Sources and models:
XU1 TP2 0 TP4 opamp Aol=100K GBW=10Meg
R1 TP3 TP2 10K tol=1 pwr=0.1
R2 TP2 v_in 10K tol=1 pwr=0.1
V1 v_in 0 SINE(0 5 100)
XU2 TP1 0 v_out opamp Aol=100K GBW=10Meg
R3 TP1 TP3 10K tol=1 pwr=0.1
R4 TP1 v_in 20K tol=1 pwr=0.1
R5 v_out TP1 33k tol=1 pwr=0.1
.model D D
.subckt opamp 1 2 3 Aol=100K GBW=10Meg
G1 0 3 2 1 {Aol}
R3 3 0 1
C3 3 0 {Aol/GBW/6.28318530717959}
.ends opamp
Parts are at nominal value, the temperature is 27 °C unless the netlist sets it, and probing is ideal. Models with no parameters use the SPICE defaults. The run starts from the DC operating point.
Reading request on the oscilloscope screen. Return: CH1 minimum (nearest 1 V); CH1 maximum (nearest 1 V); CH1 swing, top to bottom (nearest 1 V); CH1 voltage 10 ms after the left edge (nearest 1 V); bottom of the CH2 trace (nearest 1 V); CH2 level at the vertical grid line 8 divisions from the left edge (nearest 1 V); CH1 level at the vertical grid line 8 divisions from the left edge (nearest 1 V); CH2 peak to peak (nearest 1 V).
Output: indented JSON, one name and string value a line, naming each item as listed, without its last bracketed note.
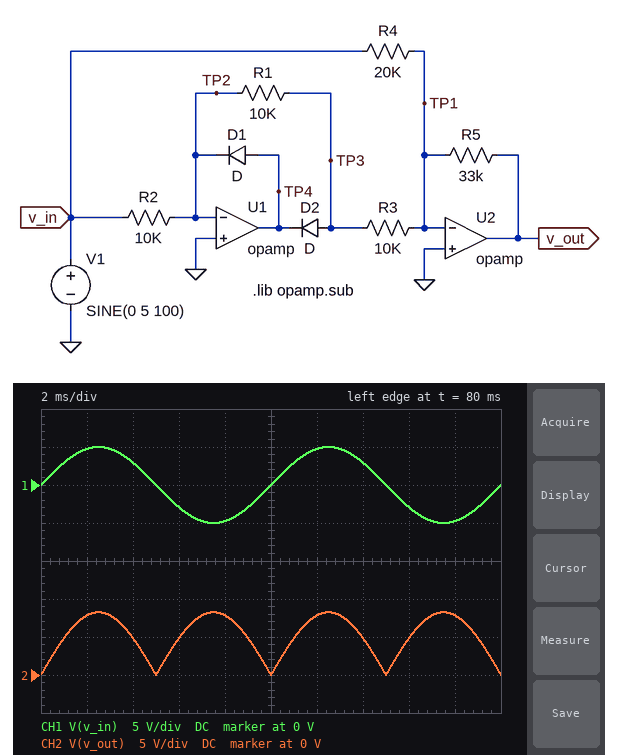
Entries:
{
  "CH1 minimum": "-5 V",
  "CH1 maximum": "5 V",
  "CH1 swing, top to bottom": "10 V",
  "CH1 voltage 10 ms after the left edge": "0 V",
  "bottom of the CH2 trace": "0 V",
  "CH2 level at the vertical grid line 8 divisions from the left edge": "5 V",
  "CH1 level at the vertical grid line 8 divisions from the left edge": "-3 V",
  "CH2 peak to peak": "8 V"
}
